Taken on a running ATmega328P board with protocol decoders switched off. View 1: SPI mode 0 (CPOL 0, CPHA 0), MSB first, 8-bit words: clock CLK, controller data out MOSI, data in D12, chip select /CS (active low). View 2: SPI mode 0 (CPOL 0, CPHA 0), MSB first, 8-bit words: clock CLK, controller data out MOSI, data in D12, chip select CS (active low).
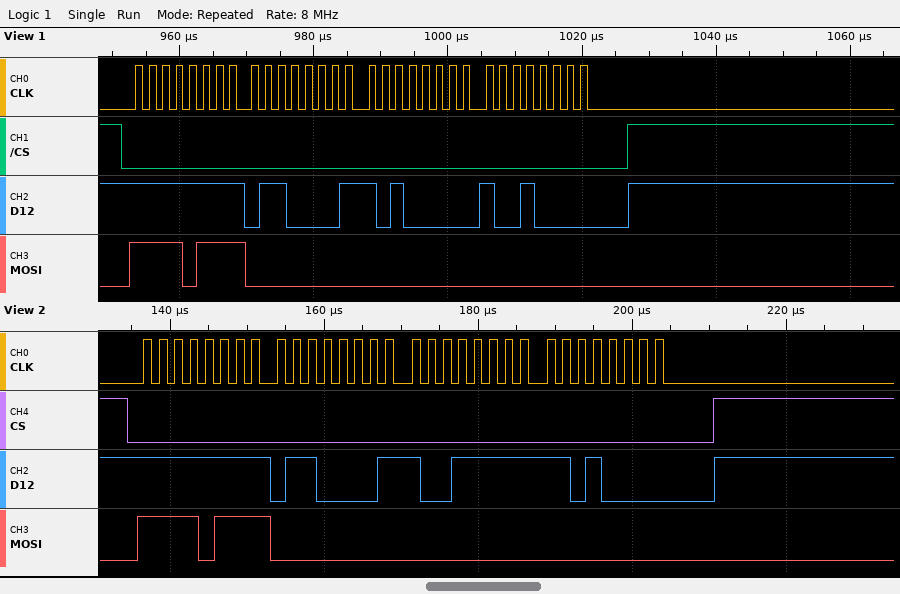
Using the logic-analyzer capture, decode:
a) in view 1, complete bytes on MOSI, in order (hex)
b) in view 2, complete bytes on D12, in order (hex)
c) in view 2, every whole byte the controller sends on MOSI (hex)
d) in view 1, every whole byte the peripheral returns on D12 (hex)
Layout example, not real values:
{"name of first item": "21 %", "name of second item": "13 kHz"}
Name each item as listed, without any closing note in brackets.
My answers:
{"in view 1, complete bytes on MOSI, in order": "F7 00 00 00", "in view 2, complete bytes on D12, in order": "FF 61 9F D0", "in view 2, every whole byte the controller sends on MOSI": "F7 00 00 00", "in view 1, every whole byte the peripheral returns on D12": "FF 61 A0 90"}
